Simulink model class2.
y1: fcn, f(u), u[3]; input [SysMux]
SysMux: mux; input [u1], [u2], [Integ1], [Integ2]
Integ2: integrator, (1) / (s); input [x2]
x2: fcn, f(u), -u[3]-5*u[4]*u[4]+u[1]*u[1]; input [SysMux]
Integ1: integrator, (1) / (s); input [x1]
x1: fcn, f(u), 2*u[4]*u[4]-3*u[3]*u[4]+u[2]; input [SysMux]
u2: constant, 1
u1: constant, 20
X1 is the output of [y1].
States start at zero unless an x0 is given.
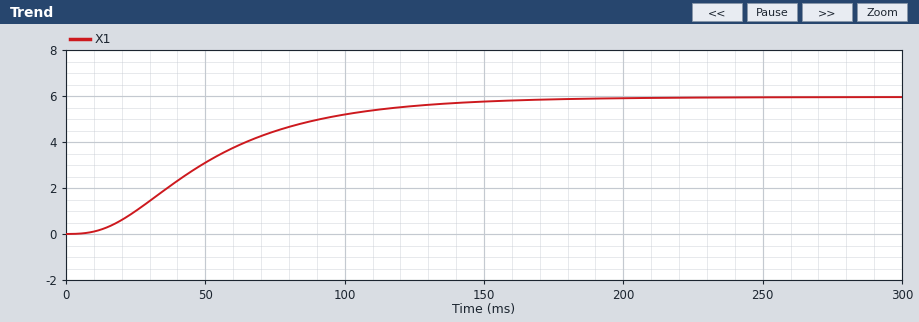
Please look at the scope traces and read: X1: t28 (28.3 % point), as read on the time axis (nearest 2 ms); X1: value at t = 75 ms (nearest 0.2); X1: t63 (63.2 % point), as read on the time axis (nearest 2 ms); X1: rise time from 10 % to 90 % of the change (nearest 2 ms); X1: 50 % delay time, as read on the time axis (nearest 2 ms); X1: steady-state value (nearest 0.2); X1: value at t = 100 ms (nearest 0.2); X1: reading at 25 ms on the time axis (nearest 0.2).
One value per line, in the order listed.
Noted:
32 ms
4.4
60 ms
90 ms
48 ms
6.0
5.2
1.0
